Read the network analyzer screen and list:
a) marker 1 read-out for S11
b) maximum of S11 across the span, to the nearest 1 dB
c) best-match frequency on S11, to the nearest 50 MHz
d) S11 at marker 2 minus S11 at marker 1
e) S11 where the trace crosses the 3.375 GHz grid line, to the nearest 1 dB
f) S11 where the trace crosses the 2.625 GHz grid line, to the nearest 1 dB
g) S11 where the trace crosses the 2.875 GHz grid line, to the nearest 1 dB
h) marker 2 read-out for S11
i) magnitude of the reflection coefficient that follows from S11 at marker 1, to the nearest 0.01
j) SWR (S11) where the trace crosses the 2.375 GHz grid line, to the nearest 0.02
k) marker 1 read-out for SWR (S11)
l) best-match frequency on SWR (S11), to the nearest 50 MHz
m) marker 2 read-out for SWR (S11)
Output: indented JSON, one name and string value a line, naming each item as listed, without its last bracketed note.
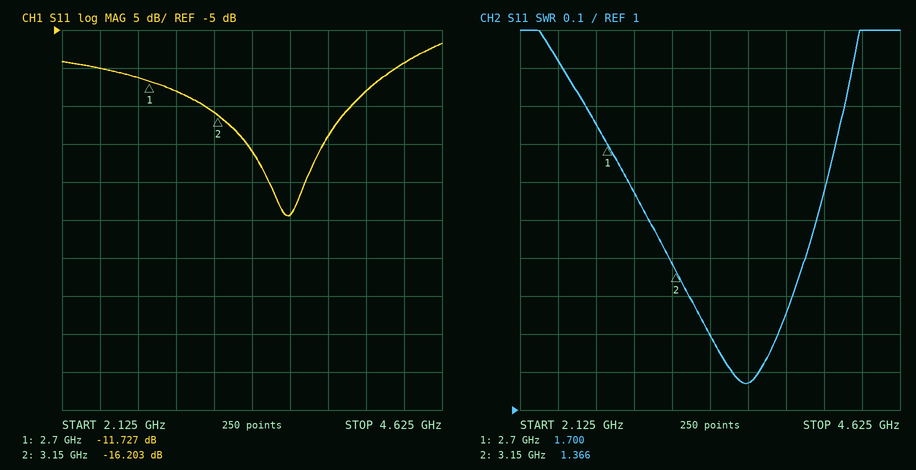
{
  "marker 1 read-out for S11": "-11.727 dB",
  "maximum of S11 across the span, to the nearest 1 dB": "-7 dB",
  "best-match frequency on S11, to the nearest 50 MHz": "3.60 GHz",
  "S11 at marker 2 minus S11 at marker 1": "-4.476 dB",
  "S11 where the trace crosses the 3.375 GHz grid line, to the nearest 1 dB": "-21 dB",
  "S11 where the trace crosses the 2.625 GHz grid line, to the nearest 1 dB": "-11 dB",
  "S11 where the trace crosses the 2.875 GHz grid line, to the nearest 1 dB": "-13 dB",
  "marker 2 read-out for S11": "-16.203 dB",
  "magnitude of the reflection coefficient that follows from S11 at marker 1, to the nearest 0.01": "0.26",
  "SWR (S11) where the trace crosses the 2.375 GHz grid line, to the nearest 0.02": "1.92",
  "marker 1 read-out for SWR": "1.700",
  "best-match frequency on SWR (S11), to the nearest 50 MHz": "3.60 GHz",
  "marker 2 read-out for SWR": "1.366"
}
